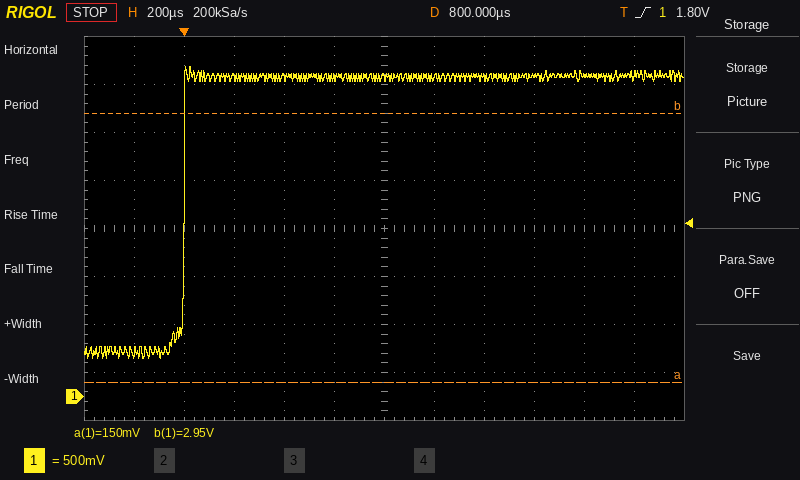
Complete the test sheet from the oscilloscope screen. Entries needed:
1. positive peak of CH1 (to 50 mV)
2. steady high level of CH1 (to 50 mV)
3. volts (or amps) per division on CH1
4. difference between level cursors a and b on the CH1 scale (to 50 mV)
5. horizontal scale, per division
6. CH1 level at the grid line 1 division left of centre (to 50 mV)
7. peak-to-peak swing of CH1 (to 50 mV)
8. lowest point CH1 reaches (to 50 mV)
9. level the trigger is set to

3.45 V
3.35 V
500 mV
2.80 V
200 µs
3.30 V
3.05 V
400 mV
1.80 V
